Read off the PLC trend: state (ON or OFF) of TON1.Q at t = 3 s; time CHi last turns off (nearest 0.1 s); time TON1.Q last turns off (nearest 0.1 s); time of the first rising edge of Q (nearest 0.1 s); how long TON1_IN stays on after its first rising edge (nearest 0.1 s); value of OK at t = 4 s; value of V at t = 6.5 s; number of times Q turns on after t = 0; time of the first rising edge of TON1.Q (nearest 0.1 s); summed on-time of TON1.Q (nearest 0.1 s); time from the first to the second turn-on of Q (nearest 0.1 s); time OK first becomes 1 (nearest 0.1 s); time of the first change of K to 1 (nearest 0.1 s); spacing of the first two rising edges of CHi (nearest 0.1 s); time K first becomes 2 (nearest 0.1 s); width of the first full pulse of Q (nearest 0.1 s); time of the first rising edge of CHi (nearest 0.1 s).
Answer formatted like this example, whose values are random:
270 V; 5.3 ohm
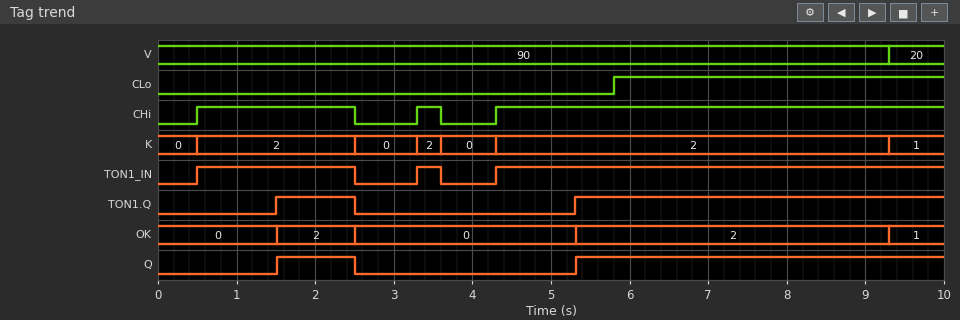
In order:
OFF; 3.6 s; 2.5 s; 1.5 s; 2.0 s; 0; 90; 2; 1.5 s; 5.7 s; 3.8 s; 9.3 s; 9.3 s; 2.8 s; 0.5 s; 1.0 s; 0.5 s
